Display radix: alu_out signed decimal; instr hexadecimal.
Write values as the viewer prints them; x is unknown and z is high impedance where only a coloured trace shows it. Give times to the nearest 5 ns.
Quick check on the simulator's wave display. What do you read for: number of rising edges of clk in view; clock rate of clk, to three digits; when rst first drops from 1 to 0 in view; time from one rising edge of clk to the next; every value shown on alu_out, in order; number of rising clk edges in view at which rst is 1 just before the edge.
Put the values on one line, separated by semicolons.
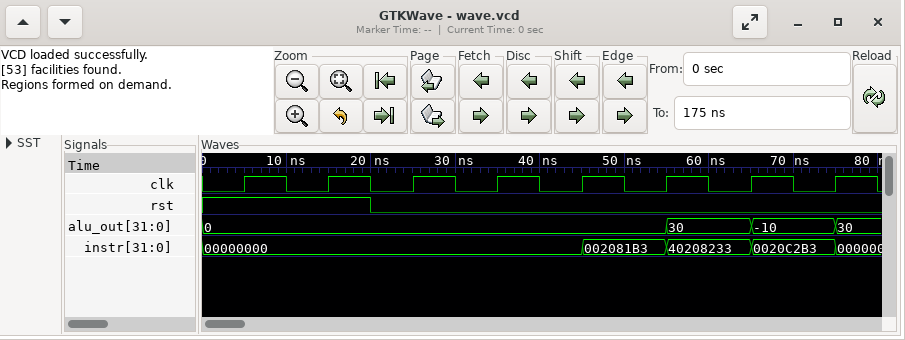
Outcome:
8; 100 MHz; 20 ns; 10 ns; 0, 30, -10, 30; 2
